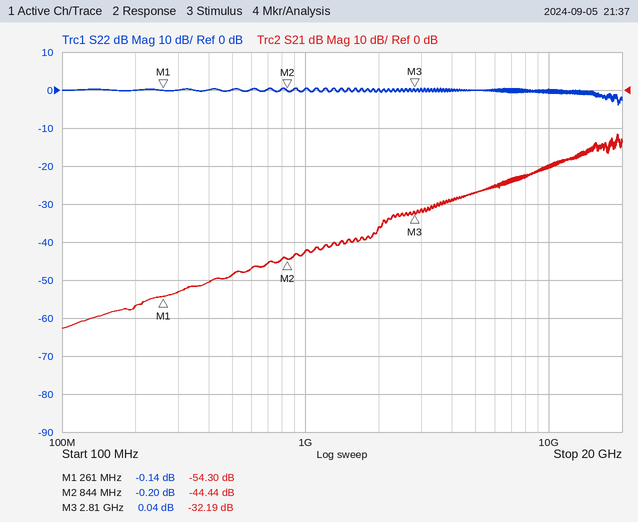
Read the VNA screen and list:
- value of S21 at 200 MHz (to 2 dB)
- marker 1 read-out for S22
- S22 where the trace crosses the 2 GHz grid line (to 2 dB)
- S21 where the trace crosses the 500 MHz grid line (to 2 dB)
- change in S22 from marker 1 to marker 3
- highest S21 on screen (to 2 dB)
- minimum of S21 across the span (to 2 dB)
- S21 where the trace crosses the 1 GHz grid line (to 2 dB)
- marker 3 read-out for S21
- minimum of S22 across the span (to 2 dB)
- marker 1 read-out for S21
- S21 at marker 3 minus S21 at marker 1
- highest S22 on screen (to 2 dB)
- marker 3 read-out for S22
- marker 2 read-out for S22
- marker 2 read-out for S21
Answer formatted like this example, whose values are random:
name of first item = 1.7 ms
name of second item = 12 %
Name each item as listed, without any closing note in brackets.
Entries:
value of S21 at 200 MHz = -56 dB
marker 1 read-out for S22 = -0.14 dB
S22 where the trace crosses the 2 GHz grid line = 0 dB
S21 where the trace crosses the 500 MHz grid line = -48 dB
change in S22 from marker 1 to marker 3 = 0.18 dB
highest S21 on screen = -12 dB
minimum of S21 across the span = -62 dB
S21 where the trace crosses the 1 GHz grid line = -42 dB
marker 3 read-out for S21 = -32.19 dB
minimum of S22 across the span = -4 dB
marker 1 read-out for S21 = -54.30 dB
S21 at marker 3 minus S21 at marker 1 = 22.11 dB
highest S22 on screen = 0 dB
marker 3 read-out for S22 = 0.04 dB
marker 2 read-out for S22 = -0.20 dB
marker 2 read-out for S21 = -44.44 dB
